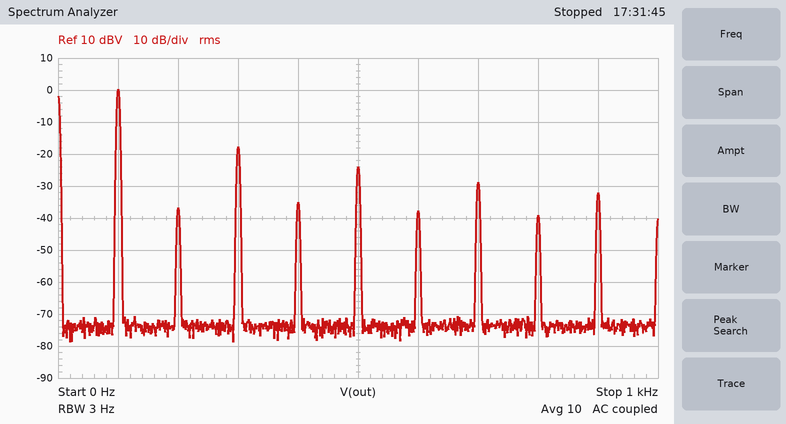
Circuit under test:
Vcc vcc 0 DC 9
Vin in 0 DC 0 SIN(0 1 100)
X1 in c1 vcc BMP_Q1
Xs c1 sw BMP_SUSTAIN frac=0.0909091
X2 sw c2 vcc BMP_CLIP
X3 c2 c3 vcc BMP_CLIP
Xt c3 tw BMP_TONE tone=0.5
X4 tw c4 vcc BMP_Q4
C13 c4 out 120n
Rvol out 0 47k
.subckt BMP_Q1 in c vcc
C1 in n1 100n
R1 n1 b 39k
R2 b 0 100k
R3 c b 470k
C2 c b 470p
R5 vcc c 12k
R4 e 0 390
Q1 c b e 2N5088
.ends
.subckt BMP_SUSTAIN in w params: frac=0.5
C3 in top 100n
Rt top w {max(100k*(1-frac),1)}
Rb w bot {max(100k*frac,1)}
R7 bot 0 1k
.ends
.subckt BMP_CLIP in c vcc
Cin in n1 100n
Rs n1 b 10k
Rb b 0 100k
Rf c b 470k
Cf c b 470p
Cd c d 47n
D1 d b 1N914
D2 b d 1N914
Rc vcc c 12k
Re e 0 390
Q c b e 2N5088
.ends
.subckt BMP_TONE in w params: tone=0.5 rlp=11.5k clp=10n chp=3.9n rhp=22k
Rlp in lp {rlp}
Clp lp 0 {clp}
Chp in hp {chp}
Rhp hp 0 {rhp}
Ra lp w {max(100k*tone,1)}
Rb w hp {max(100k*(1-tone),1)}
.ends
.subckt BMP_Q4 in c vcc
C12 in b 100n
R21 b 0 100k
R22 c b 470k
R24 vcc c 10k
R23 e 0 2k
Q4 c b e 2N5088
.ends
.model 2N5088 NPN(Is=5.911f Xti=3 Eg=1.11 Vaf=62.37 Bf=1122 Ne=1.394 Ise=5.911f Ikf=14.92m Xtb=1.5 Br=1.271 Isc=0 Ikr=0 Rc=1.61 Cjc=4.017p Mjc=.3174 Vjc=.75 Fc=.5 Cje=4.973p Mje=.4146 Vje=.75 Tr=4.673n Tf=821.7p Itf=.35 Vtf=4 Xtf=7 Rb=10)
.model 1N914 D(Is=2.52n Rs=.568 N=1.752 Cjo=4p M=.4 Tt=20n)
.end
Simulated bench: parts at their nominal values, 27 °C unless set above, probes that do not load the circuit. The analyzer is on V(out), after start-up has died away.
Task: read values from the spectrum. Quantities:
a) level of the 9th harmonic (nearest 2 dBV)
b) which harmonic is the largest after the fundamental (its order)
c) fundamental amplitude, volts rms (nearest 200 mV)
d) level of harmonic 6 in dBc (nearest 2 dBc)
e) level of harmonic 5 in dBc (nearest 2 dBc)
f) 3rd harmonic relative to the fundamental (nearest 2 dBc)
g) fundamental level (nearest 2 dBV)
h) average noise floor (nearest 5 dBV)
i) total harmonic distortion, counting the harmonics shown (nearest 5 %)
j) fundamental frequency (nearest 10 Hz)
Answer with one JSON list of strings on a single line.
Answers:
["-32 dBV", "3", "1.0 V", "-38 dBc", "-24 dBc", "-18 dBc", "0 dBV", "-75 dBV", "15 %", "100 Hz"]
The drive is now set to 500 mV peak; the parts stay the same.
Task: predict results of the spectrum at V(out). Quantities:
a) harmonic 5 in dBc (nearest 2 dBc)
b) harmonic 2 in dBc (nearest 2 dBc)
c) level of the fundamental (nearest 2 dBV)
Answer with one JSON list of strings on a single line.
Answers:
["-22 dBc", "-46 dBc", "-2 dBV"]
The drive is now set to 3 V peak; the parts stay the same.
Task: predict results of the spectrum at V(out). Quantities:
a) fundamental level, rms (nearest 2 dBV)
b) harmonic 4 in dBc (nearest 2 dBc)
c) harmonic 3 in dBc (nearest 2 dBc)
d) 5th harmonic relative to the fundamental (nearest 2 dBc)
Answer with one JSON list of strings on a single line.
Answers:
["0 dBV", "-26 dBc", "-26 dBc", "-28 dBc"]
